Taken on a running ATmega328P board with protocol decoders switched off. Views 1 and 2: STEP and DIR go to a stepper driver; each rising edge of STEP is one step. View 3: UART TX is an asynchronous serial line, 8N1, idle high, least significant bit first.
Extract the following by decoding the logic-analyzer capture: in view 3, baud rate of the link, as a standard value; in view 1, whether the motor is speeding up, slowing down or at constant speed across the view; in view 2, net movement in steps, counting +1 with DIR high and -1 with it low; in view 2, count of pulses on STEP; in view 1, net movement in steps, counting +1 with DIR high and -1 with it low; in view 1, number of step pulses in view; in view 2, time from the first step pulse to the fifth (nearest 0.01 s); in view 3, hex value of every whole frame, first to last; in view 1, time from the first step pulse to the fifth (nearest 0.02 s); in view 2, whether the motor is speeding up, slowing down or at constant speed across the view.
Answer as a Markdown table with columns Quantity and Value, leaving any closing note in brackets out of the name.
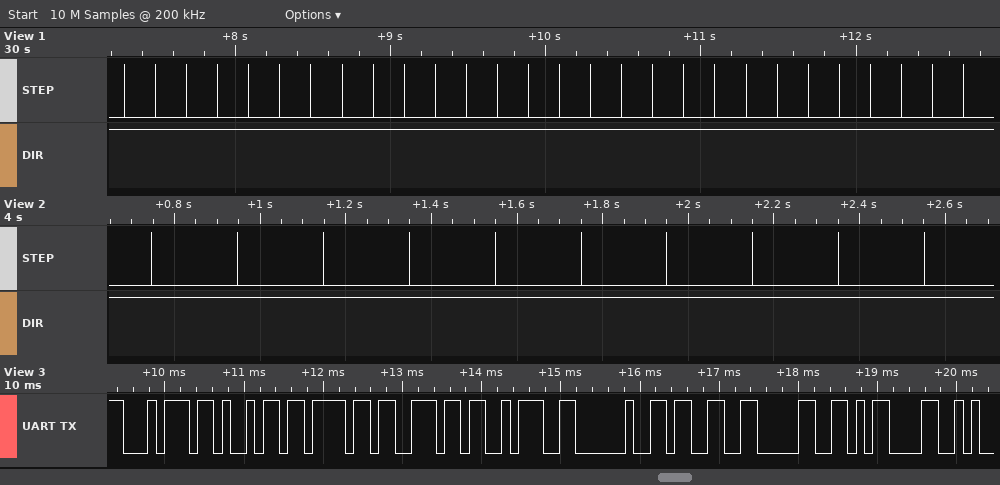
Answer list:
| Quantity | Value |
|---|---|
| in view 3, baud rate of the link, as a standard value | 9600 baud |
| in view 1, whether the motor is speeding up, slowing down or at constant speed across the view | constant speed |
| in view 2, net movement in steps, counting +1 with DIR high and -1 with it low | +10 |
| in view 2, count of pulses on STEP | 10 |
| in view 1, net movement in steps, counting +1 with DIR high and -1 with it low | +28 |
| in view 1, number of step pulses in view | 28 |
| in view 2, time from the first step pulse to the fifth | 0.80 s |
| in view 3, hex value of every whole frame, first to last | 74 69 6F 6E 3A 20 33 30 0D |
| in view 1, time from the first step pulse to the fifth | 0.80 s |
| in view 2, whether the motor is speeding up, slowing down or at constant speed across the view | constant speed |
